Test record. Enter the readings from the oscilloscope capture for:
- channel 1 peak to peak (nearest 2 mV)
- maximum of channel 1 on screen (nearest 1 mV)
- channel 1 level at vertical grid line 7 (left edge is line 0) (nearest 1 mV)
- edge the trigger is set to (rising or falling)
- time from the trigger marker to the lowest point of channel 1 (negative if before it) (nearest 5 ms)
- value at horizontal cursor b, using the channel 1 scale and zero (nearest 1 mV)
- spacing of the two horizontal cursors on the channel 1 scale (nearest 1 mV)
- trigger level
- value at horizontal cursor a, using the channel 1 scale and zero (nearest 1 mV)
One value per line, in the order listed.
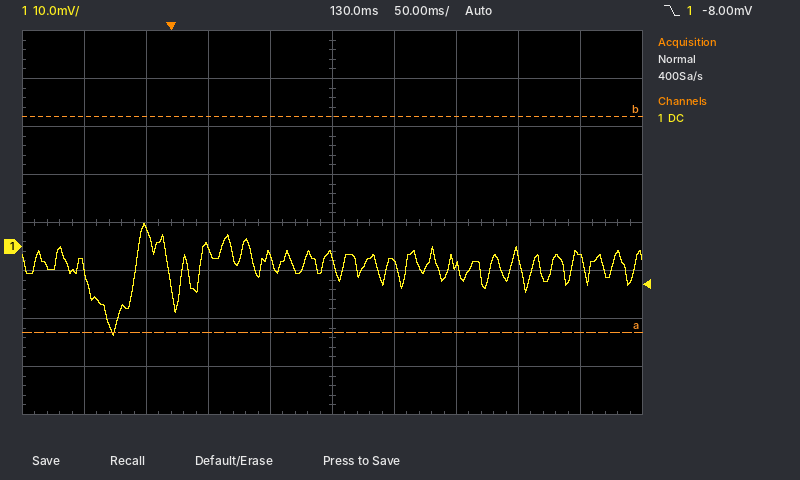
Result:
24 mV
5 mV
-4 mV
falling
-45 ms
27 mV
45 mV
-8.00 mV
-18 mV
